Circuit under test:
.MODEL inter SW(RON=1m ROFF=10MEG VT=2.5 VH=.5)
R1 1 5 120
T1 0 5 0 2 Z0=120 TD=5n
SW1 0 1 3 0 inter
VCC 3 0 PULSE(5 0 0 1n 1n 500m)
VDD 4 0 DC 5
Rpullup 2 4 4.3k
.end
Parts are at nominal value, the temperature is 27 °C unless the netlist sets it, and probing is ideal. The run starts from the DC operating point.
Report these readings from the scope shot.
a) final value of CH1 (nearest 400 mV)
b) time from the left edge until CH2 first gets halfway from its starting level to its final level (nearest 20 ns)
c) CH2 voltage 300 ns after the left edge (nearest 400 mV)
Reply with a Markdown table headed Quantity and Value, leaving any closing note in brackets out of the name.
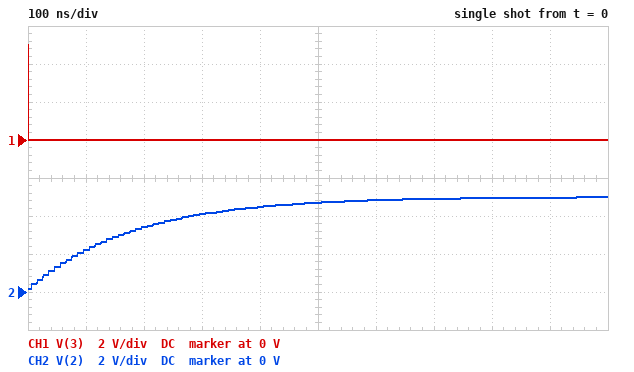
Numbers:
| Quantity | Value |
|---|---|
| final value of CH1 | 0 V |
| time from the left edge until CH2 first gets halfway from its starting level to its final level | 120 ns |
| CH2 voltage 300 ns after the left edge | 4.0 V |
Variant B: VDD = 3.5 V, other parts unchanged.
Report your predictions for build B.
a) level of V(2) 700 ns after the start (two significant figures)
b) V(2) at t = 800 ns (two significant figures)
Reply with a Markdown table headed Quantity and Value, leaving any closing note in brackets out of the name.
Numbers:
| Quantity | Value |
|---|---|
| level of V(2) 700 ns after the start | 3.4 V |
| V(2) at t = 800 ns | 3.5 V |
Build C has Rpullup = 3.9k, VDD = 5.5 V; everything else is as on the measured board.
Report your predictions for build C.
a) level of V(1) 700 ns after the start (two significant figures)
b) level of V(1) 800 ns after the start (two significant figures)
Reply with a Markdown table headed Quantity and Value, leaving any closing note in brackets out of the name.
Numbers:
| Quantity | Value |
|---|---|
| level of V(1) 700 ns after the start | 5.4 V |
| level of V(1) 800 ns after the start | 5.5 V |
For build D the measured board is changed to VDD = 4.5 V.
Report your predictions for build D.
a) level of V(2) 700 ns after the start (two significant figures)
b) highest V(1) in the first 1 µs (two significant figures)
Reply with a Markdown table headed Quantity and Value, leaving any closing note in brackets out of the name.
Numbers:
| Quantity | Value |
|---|---|
| level of V(2) 700 ns after the start | 4.4 V |
| highest V(1) in the first 1 µs | 4.5 V |
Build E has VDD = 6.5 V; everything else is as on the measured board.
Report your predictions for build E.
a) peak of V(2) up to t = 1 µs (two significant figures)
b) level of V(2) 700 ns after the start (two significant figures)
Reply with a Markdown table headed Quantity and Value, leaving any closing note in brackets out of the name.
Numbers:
| Quantity | Value |
|---|---|
| peak of V(2) up to t = 1 µs | 6.5 V |
| level of V(2) 700 ns after the start | 6.4 V |
